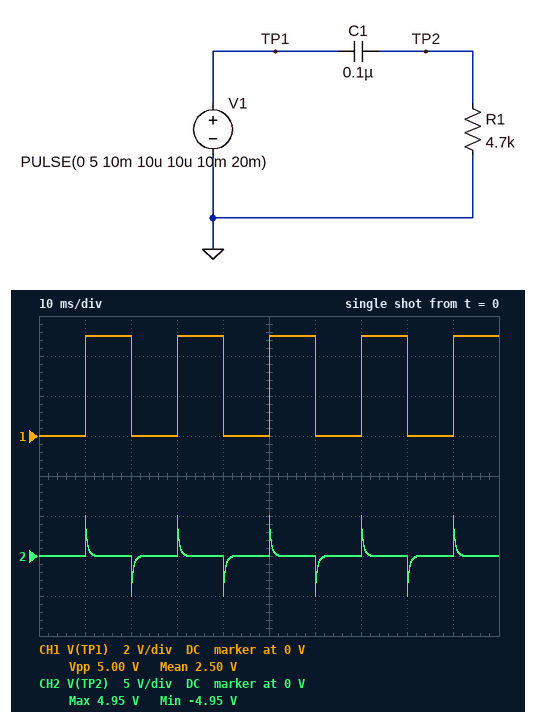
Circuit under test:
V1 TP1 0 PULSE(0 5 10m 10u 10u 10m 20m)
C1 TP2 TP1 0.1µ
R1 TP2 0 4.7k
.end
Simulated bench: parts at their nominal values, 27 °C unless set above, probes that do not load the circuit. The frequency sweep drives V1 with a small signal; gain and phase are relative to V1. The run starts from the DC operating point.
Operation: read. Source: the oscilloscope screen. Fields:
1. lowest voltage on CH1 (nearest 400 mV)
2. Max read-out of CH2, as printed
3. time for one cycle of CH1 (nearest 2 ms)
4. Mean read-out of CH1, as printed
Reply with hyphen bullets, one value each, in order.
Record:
- 0 V
- 4.95 V
- 20 ms
- 2.50 V
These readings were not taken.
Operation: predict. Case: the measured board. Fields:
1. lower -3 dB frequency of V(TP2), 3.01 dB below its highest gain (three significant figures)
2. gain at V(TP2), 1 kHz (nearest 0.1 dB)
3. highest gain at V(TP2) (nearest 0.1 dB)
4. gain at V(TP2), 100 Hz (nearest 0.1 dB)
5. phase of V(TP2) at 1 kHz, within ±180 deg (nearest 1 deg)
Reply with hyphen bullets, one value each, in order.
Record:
- 339 Hz
- -0.5 dB
- 0 dB
- -11.0 dB
- 19 deg
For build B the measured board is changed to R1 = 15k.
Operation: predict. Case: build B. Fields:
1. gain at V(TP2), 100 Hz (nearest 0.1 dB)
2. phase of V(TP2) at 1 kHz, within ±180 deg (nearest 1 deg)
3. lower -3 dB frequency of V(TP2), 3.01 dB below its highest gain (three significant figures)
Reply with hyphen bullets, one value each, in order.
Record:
- -3.3 dB
- 6 deg
- 106 Hz
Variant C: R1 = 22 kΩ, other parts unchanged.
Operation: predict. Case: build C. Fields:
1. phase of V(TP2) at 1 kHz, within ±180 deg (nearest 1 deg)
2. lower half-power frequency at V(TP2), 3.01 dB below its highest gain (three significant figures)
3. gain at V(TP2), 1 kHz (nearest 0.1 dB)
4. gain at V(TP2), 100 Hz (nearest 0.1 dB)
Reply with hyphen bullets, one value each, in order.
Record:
- 4 deg
- 72.3 Hz
- 0 dB
- -1.8 dB
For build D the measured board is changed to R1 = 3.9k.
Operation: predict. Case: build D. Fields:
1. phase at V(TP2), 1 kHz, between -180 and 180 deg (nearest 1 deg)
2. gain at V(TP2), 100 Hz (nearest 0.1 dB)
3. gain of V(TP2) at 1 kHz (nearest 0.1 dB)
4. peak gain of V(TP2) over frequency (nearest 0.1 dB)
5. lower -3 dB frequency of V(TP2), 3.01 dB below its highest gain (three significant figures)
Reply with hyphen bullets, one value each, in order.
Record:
- 22 deg
- -12.5 dB
- -0.7 dB
- 0 dB
- 408 Hz
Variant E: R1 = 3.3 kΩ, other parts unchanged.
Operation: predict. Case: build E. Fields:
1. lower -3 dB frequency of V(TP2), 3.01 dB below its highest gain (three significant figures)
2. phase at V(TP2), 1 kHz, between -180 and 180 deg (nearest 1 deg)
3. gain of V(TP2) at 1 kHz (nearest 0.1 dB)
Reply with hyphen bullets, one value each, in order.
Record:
- 482 Hz
- 26 deg
- -0.9 dB
